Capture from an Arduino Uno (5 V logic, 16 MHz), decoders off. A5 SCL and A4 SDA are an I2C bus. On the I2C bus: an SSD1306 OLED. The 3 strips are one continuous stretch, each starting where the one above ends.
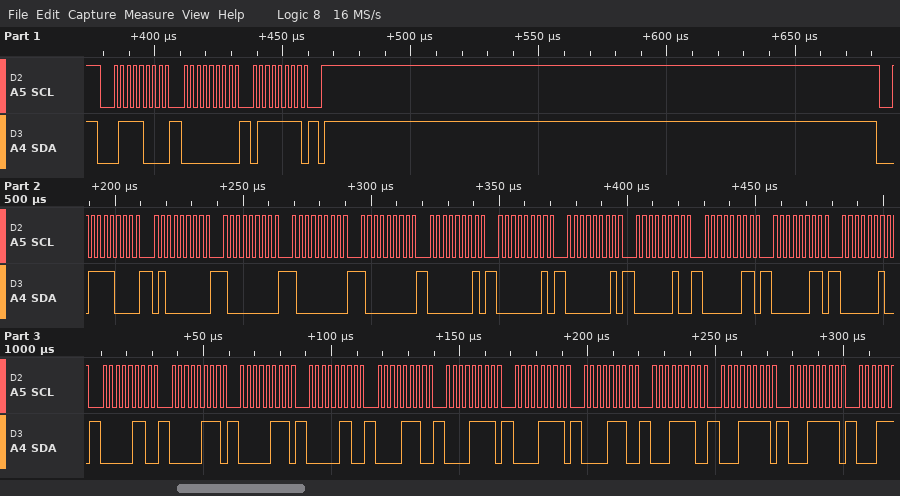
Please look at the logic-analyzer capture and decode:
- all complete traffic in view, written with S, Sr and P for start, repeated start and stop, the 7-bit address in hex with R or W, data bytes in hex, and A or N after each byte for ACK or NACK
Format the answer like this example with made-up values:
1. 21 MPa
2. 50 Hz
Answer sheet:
1. S 3CW A 00 A 7F A P S 3CW A 40 A 80 A 80 A 80 A 01 A 01 A 01 A 02 A 03 A 03 A 02 A 06 A 07 A 07 A 06 A 0E A 0F A 0F A 0E A 1E A 1F A 1F A
